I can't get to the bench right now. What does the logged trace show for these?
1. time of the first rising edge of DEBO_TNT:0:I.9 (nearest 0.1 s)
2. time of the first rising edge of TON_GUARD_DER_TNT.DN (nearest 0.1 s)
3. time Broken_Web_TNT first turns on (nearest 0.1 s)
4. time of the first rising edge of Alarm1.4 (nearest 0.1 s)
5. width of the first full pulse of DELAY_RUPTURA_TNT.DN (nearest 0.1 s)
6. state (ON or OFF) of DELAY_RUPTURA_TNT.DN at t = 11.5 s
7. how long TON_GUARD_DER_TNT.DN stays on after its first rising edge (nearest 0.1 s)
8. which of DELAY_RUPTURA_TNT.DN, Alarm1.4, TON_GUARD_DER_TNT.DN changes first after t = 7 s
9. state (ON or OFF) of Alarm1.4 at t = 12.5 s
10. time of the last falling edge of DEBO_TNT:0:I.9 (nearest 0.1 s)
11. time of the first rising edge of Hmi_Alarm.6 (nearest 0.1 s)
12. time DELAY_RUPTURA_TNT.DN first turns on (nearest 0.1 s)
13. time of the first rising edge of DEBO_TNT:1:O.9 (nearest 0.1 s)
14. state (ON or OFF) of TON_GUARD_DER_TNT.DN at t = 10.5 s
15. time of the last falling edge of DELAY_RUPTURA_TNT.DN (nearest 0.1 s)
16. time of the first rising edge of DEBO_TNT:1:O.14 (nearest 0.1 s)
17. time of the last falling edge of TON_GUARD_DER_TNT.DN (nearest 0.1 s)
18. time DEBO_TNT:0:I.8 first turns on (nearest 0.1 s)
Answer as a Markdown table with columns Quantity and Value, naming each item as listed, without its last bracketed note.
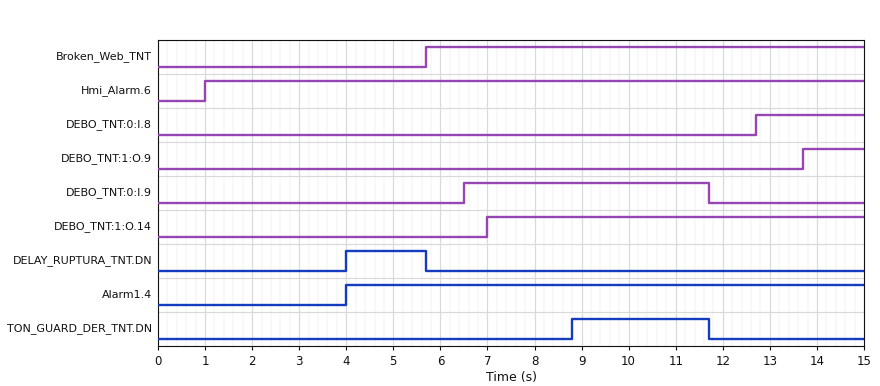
| Quantity | Value |
|---|---|
| time of the first rising edge of DEBO_TNT:0:I.9 | 6.5 s |
| time of the first rising edge of TON_GUARD_DER_TNT.DN | 8.8 s |
| time Broken_Web_TNT first turns on | 5.7 s |
| time of the first rising edge of Alarm1.4 | 4.0 s |
| width of the first full pulse of DELAY_RUPTURA_TNT.DN | 1.7 s |
| state (ON or OFF) of DELAY_RUPTURA_TNT.DN at t = 11.5 s | OFF |
| how long TON_GUARD_DER_TNT.DN stays on after its first rising edge | 2.9 s |
| which of DELAY_RUPTURA_TNT.DN, Alarm1.4, TON_GUARD_DER_TNT.DN changes first after t = 7 s | TON_GUARD_DER_TNT.DN |
| state (ON or OFF) of Alarm1.4 at t = 12.5 s | ON |
| time of the last falling edge of DEBO_TNT:0:I.9 | 11.7 s |
| time of the first rising edge of Hmi_Alarm.6 | 1.0 s |
| time DELAY_RUPTURA_TNT.DN first turns on | 4.0 s |
| time of the first rising edge of DEBO_TNT:1:O.9 | 13.7 s |
| state (ON or OFF) of TON_GUARD_DER_TNT.DN at t = 10.5 s | ON |
| time of the last falling edge of DELAY_RUPTURA_TNT.DN | 5.7 s |
| time of the first rising edge of DEBO_TNT:1:O.14 | 7.0 s |
| time of the last falling edge of TON_GUARD_DER_TNT.DN | 11.7 s |
| time DEBO_TNT:0:I.8 first turns on | 12.7 s |
